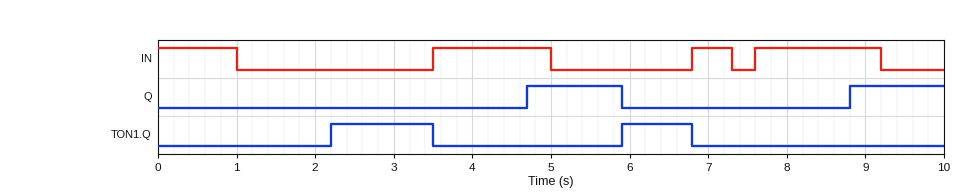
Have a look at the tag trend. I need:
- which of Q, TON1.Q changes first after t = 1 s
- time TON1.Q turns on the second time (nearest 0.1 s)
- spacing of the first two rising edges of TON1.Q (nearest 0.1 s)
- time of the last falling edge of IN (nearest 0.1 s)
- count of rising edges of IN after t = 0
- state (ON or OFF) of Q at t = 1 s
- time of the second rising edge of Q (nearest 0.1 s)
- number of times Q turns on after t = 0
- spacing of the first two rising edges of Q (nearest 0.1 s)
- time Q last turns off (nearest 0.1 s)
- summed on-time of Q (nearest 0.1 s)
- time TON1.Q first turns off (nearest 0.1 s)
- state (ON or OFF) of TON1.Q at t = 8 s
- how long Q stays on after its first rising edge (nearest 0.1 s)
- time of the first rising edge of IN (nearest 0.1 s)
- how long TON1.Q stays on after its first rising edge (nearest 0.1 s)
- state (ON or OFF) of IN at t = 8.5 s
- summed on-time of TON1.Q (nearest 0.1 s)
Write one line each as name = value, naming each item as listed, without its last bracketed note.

which of Q, TON1.Q changes first after t = 1 s = TON1.Q
time TON1.Q turns on the second time = 5.9 s
spacing of the first two rising edges of TON1.Q = 3.7 s
time of the last falling edge of IN = 9.2 s
count of rising edges of IN after t = 0 = 3
state (ON or OFF) of Q at t = 1 s = OFF
time of the second rising edge of Q = 8.8 s
number of times Q turns on after t = 0 = 2
spacing of the first two rising edges of Q = 4.1 s
time Q last turns off = 5.9 s
summed on-time of Q = 2.4 s
time TON1.Q first turns off = 3.5 s
state (ON or OFF) of TON1.Q at t = 8 s = OFF
how long Q stays on after its first rising edge = 1.2 s
time of the first rising edge of IN = 3.5 s
how long TON1.Q stays on after its first rising edge = 1.3 s
state (ON or OFF) of IN at t = 8.5 s = ON
summed on-time of TON1.Q = 2.2 s
